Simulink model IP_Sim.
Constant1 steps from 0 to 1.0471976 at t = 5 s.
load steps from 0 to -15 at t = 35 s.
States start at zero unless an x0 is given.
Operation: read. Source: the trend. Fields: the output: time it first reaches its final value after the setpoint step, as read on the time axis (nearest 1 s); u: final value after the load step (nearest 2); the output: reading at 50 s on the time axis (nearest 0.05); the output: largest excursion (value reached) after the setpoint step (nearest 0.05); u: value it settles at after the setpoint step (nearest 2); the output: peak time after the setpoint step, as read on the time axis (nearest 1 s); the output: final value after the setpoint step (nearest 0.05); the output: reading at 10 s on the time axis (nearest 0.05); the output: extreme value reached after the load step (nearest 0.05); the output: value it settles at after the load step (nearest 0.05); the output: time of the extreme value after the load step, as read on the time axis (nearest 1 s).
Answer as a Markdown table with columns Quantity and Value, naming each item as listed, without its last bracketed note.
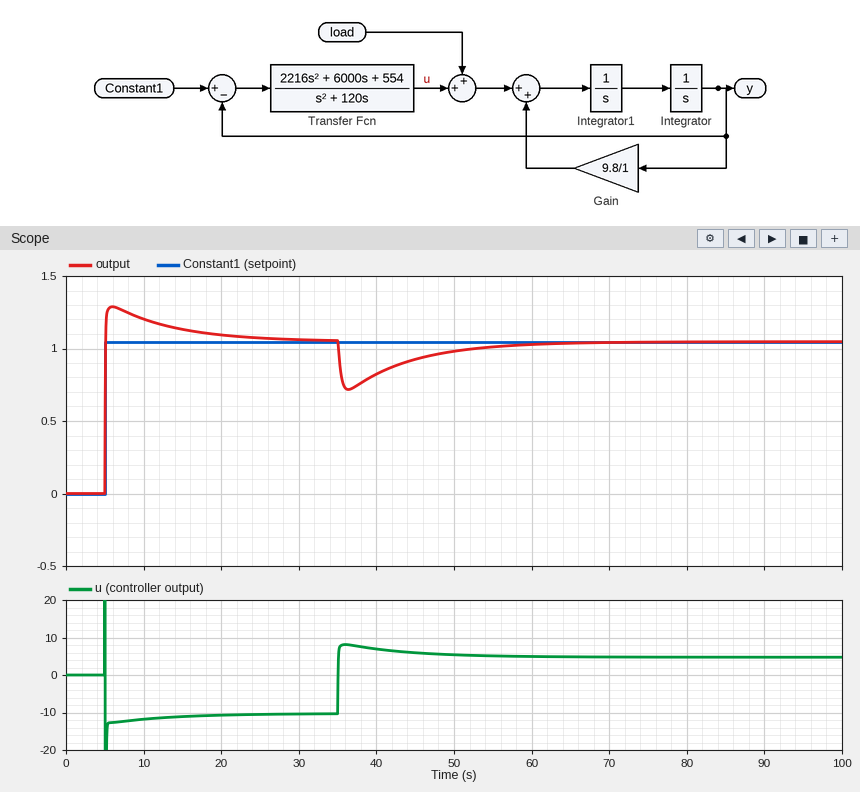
| Quantity | Value |
|---|---|
| the output: time it first reaches its final value after the setpoint step, as read on the time axis | 5 s |
| u: final value after the load step | 4 |
| the output: reading at 50 s on the time axis | 1.00 |
| the output: largest excursion (value reached) after the setpoint step | 1.30 |
| u: value it settles at after the setpoint step | -10 |
| the output: peak time after the setpoint step, as read on the time axis | 6 s |
| the output: final value after the setpoint step | 1.05 |
| the output: reading at 10 s on the time axis | 1.20 |
| the output: extreme value reached after the load step | 0.70 |
| the output: value it settles at after the load step | 1.05 |
| the output: time of the extreme value after the load step, as read on the time axis | 36 s |
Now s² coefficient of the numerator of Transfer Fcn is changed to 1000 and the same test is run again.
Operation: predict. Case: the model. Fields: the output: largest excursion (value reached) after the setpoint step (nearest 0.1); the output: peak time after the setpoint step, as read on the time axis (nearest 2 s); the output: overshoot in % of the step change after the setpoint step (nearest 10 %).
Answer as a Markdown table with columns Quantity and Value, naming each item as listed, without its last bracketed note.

| Quantity | Value |
|---|---|
| the output: largest excursion (value reached) after the setpoint step | 1.5 |
| the output: peak time after the setpoint step, as read on the time axis | 6 s |
| the output: overshoot in % of the step change after the setpoint step | 50 % |
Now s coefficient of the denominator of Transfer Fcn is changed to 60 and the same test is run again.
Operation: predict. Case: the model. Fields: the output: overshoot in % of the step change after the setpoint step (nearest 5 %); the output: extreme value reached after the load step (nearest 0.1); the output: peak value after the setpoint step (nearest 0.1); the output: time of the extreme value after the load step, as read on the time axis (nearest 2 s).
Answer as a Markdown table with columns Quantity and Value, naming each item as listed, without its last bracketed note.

| Quantity | Value |
|---|---|
| the output: overshoot in % of the step change after the setpoint step | 15 % |
| the output: extreme value reached after the load step | 0.9 |
| the output: peak value after the setpoint step | 1.2 |
| the output: time of the extreme value after the load step, as read on the time axis | 36 s |
